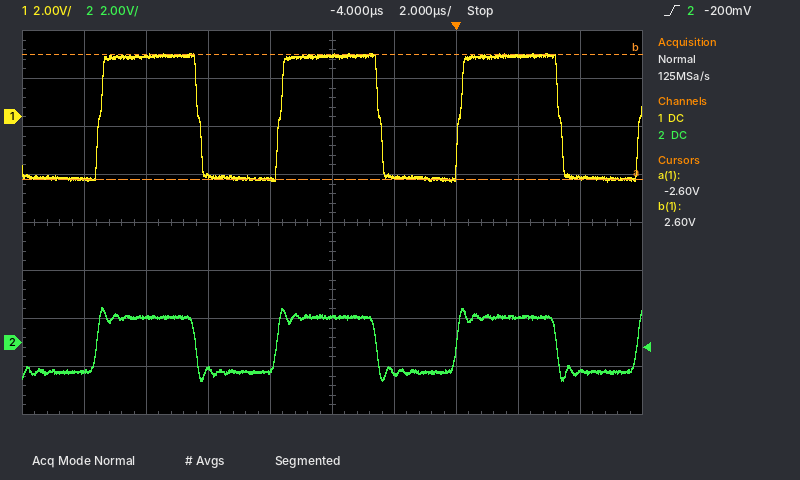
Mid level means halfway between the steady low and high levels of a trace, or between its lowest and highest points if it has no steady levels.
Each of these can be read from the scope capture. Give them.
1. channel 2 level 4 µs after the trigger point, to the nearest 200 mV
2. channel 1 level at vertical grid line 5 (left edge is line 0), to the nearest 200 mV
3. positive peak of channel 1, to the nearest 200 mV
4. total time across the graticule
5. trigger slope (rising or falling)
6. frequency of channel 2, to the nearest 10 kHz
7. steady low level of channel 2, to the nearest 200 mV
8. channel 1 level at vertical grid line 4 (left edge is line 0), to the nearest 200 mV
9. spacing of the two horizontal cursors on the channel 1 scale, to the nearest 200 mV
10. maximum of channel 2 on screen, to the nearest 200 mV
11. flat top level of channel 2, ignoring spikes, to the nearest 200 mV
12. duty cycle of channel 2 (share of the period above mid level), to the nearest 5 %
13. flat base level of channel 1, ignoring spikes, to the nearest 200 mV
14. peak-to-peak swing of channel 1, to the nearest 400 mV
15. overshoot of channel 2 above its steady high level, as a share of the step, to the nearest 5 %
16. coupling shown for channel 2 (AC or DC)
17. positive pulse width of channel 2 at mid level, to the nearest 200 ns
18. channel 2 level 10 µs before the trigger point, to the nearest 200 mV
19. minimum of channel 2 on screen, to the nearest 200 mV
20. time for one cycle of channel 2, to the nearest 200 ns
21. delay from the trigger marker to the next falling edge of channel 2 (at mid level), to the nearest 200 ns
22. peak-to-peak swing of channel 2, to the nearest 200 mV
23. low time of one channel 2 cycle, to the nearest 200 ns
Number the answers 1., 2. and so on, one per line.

1. -1.2 V
2. 2.6 V
3. 2.6 V
4. 20 µs
5. rising
6. 170 kHz
7. -1.2 V
8. -2.6 V
9. 5.2 V
10. 1.4 V
11. 1.0 V
12. 55 %
13. -2.6 V
14. 5.2 V
15. 15 %
16. DC
17. 3.2 µs
18. 1.0 V
19. -1.6 V
20. 5.8 µs
21. 3.2 µs
22. 3.0 V
23. 2.6 µs
